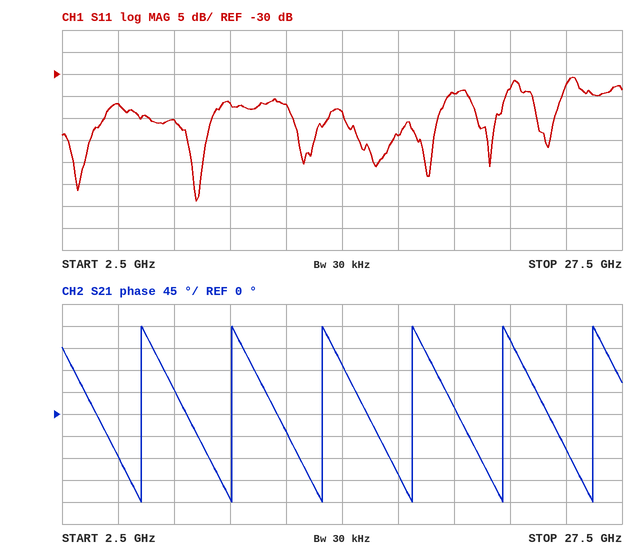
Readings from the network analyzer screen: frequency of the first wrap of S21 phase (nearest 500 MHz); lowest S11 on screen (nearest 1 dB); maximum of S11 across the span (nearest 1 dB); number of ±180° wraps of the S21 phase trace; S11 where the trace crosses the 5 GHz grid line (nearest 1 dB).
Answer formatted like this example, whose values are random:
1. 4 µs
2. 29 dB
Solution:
1. 6.0 GHz
2. -59 dB
3. -31 dB
4. 6
5. -37 dB
